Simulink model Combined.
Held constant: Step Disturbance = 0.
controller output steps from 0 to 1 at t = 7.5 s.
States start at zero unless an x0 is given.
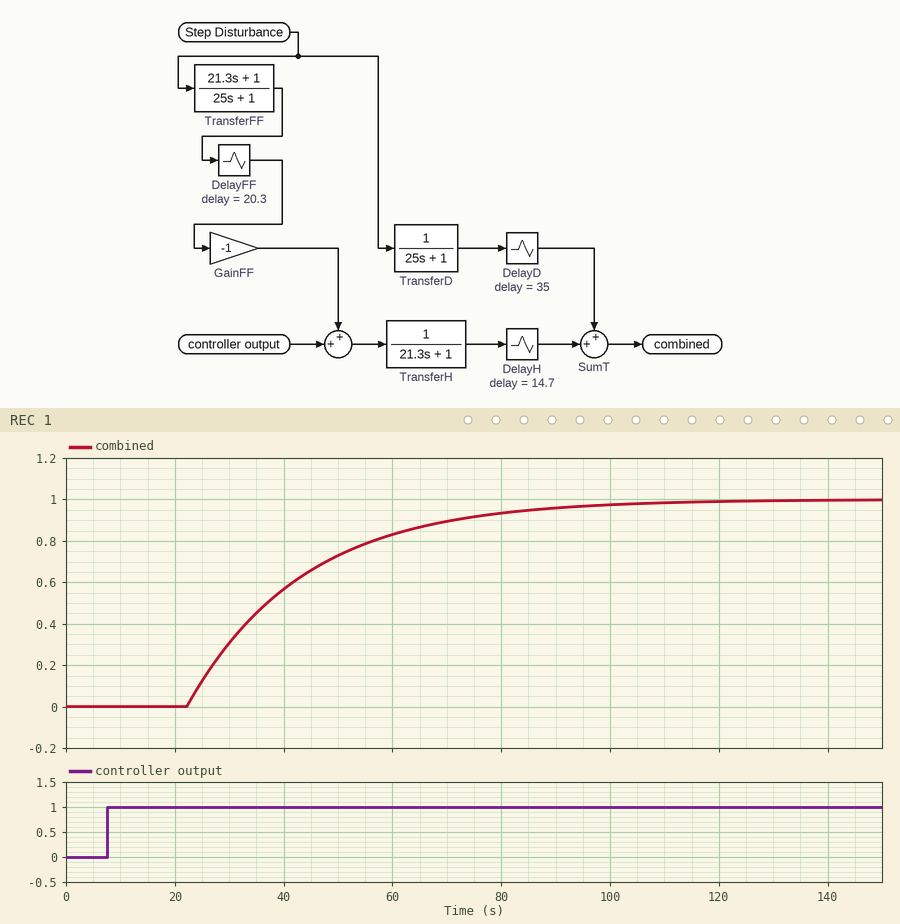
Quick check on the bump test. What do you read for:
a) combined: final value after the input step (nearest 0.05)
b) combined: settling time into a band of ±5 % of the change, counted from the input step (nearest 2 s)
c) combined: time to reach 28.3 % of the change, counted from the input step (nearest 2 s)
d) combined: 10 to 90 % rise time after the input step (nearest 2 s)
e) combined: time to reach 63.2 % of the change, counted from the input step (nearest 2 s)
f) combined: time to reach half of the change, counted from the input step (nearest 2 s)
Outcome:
1.00
78 s
22 s
46 s
36 s
30 s
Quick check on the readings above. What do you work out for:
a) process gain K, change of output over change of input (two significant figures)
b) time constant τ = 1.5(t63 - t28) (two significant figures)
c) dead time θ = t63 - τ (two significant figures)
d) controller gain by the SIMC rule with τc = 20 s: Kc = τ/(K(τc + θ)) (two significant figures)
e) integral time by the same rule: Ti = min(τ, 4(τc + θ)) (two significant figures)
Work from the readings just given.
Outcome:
1.0
21 s
15 s
0.60
21 s
